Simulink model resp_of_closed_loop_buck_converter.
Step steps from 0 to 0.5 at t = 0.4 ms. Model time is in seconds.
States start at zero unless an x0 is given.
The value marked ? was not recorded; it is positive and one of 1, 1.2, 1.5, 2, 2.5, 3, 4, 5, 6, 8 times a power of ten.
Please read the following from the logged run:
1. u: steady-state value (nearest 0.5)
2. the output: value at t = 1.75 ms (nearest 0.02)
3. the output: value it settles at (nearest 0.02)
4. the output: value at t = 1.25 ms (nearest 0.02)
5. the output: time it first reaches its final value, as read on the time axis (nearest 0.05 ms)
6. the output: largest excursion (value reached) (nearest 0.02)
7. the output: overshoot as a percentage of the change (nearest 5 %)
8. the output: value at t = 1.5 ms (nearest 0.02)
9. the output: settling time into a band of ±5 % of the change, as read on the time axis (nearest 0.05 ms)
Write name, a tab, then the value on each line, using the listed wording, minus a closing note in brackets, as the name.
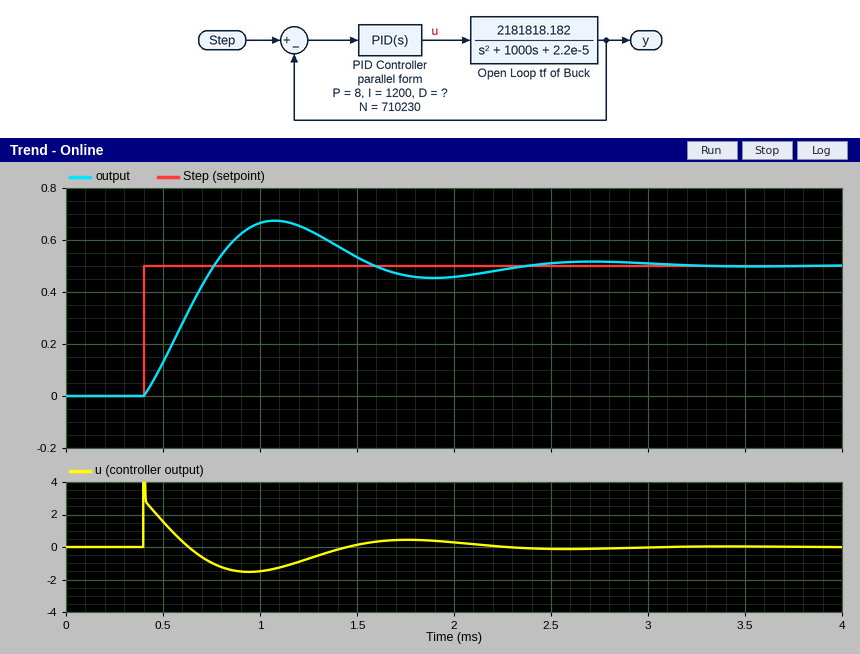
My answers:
u: steady-state value	0.0
the output: value at t = 1.75 ms	0.46
the output: value it settles at	0.50
the output: value at t = 1.25 ms	0.64
the output: time it first reaches its final value, as read on the time axis	0.75 ms
the output: largest excursion (value reached)	0.68
the output: overshoot as a percentage of the change	35 %
the output: value at t = 1.5 ms	0.54
the output: settling time into a band of ±5 % of the change, as read on the time axis	2.15 ms
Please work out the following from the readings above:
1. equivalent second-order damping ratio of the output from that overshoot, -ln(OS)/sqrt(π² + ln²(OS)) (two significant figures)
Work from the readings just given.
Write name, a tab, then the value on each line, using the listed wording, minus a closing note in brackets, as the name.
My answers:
equivalent second-order damping ratio of the output from that overshoot, -ln(OS)/sqrt(π² + ln²(OS))	0.32
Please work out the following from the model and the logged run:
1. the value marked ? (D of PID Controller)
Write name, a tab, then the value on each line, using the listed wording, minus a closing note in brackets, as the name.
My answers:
the value marked ?	0.001
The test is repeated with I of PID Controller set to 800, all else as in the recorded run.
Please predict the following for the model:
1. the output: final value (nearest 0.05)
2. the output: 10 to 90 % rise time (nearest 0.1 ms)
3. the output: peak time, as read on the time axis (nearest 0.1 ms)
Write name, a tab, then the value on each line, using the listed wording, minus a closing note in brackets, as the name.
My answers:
the output: final value	0.50
the output: 10 to 90 % rise time	0.3 ms
the output: peak time, as read on the time axis	1.1 ms
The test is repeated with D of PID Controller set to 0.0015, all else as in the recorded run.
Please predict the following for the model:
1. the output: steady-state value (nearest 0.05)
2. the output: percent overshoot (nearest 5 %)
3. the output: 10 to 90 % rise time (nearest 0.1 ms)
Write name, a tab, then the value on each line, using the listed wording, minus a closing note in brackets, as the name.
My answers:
the output: steady-state value	0.50
the output: percent overshoot	25 %
the output: 10 to 90 % rise time	0.3 ms
